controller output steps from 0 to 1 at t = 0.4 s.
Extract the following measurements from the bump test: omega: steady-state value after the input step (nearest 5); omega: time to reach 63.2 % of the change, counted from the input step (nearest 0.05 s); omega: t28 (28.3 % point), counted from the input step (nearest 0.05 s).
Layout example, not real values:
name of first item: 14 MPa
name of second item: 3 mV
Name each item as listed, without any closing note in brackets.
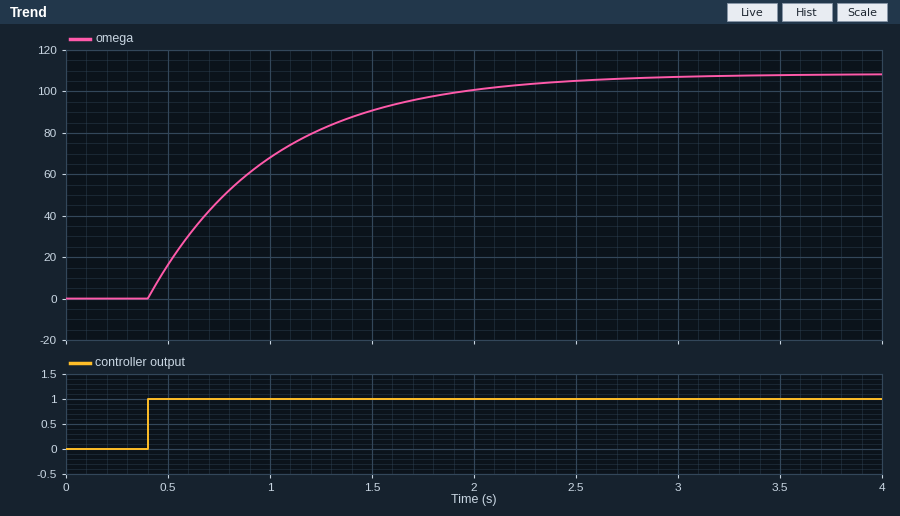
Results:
omega: steady-state value after the input step: 110
omega: time to reach 63.2 % of the change, counted from the input step: 0.60 s
omega: t28 (28.3 % point), counted from the input step: 0.20 s
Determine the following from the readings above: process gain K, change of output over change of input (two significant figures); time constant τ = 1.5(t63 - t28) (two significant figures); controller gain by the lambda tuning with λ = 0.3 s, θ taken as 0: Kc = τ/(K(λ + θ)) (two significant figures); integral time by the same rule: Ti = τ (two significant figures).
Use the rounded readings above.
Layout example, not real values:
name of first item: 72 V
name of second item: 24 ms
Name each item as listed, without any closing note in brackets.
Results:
process gain K, change of output over change of input: 110
time constant τ = 1.5(t63 - t28): 0.60 s
controller gain by the lambda tuning with λ = 0.3 s, θ taken as 0: Kc = τ/(K(λ + θ)): 0.018
integral time by the same rule: Ti = τ: 0.60 s
